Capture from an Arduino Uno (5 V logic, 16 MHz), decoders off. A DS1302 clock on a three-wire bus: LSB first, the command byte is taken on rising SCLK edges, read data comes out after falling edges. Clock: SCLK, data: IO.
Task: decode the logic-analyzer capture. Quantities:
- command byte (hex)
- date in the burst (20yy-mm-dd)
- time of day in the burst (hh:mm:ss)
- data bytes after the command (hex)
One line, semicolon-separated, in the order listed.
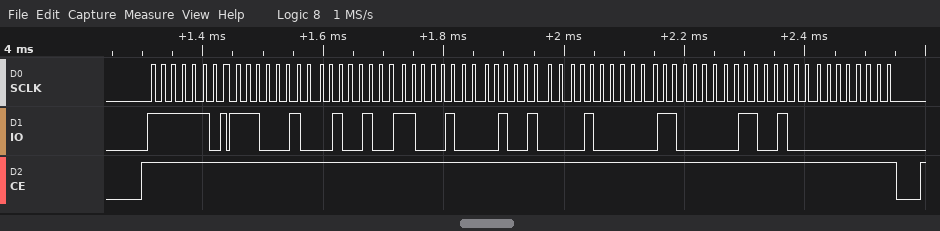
0xBF; 2026-04-24; 23:24:47; 47 24 23 24 04 06 26 00
